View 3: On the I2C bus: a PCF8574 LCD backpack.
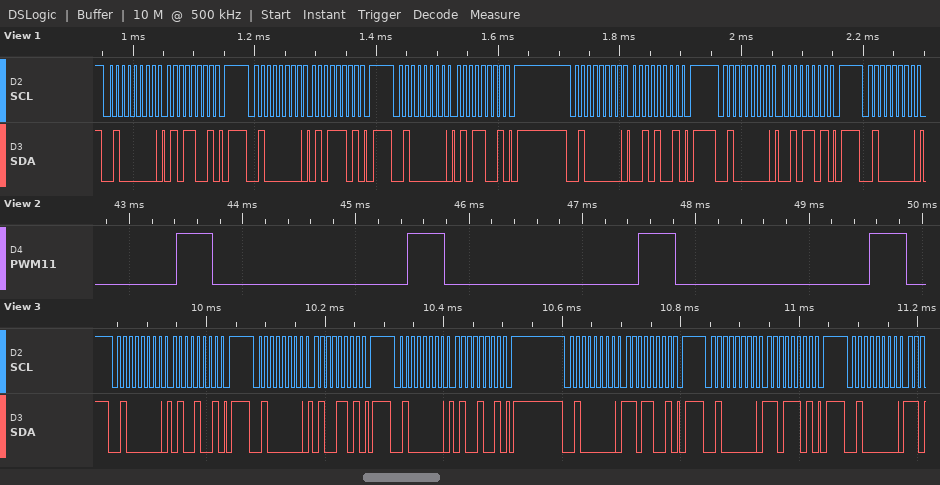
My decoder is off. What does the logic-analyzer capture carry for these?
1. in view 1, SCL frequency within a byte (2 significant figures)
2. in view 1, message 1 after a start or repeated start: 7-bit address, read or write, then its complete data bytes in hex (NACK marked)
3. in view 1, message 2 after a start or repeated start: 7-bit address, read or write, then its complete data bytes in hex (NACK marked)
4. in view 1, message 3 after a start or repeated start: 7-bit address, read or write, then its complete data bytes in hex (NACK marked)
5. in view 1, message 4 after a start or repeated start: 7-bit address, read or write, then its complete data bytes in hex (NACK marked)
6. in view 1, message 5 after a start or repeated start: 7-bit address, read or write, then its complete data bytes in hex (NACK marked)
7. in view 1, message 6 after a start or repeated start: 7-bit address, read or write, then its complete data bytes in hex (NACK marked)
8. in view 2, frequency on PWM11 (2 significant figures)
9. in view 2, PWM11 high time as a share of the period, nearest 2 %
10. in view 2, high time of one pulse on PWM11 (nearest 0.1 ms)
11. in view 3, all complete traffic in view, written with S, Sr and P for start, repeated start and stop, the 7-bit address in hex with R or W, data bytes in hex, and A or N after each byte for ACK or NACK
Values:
100 kHz
0x20 write: 59
0x20 write: 5D
0x20 write: 59
0x20 write: 29
0x20 write: 2D
0x20 write
490 Hz
16 %
0.3 ms
S 20W A 49 A P S 20W A 4D A P S 20W A 49 A P S 20W A D9 A P S 20W A DD A P S 20W A
